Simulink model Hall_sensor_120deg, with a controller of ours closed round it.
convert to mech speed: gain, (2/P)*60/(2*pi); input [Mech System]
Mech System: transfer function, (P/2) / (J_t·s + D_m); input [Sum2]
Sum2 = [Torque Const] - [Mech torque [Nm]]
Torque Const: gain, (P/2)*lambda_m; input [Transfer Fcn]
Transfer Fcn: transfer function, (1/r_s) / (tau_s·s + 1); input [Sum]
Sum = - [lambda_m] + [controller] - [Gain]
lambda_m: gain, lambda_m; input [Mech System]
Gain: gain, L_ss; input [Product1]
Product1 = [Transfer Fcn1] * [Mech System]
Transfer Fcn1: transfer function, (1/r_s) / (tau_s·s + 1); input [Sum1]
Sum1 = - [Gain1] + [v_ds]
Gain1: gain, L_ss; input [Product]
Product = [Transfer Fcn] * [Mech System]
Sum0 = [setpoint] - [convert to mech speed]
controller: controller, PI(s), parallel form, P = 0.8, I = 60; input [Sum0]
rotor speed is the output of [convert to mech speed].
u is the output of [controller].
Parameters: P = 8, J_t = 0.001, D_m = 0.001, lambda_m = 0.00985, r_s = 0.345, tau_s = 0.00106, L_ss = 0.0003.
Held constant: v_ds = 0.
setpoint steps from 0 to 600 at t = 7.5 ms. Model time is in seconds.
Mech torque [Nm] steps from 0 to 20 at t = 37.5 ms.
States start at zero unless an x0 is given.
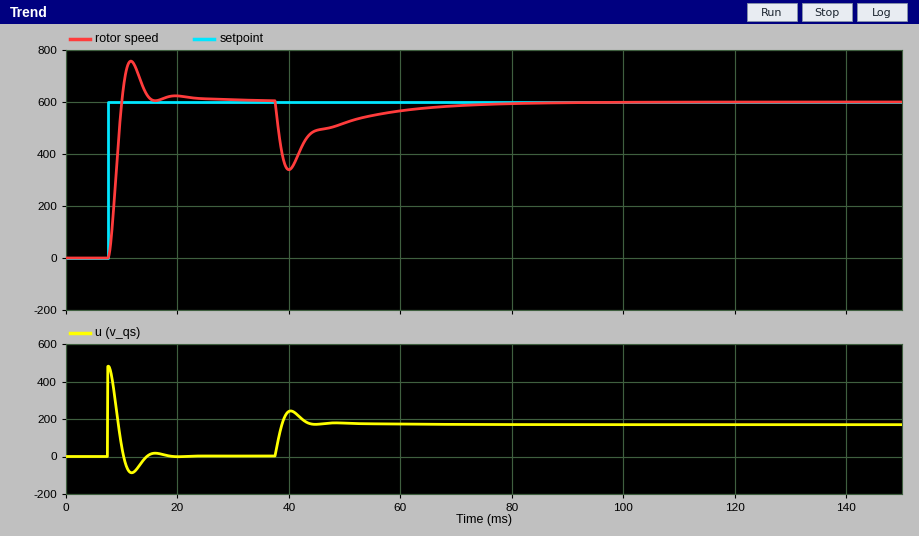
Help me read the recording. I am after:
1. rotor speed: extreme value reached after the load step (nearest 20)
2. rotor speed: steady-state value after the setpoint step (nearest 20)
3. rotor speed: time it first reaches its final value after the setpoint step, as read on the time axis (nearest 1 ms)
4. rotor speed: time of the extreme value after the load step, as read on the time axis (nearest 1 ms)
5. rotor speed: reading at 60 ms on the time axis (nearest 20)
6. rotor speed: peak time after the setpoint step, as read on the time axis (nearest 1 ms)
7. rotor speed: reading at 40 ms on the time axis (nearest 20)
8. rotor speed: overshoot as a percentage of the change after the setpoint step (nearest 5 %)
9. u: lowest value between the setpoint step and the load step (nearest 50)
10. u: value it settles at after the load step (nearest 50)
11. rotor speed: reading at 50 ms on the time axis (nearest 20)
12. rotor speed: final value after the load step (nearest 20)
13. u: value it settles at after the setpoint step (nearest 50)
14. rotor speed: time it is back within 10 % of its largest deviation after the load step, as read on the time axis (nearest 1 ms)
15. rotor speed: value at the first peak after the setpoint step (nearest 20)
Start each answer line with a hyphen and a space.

- 340
- 600
- 10 ms
- 40 ms
- 560
- 12 ms
- 340
- 25 %
- -100
- 150
- 520
- 600
- 0
- 63 ms
- 760
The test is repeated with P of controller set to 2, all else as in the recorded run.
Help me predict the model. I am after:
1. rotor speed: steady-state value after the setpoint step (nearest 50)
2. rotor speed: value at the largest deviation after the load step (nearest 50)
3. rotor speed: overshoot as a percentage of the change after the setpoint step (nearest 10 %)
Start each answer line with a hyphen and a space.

- 600
- 450
- 40 %
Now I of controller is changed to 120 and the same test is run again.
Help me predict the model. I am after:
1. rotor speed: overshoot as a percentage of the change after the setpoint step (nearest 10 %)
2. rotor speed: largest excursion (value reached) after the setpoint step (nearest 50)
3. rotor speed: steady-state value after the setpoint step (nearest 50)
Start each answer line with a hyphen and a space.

- 40 %
- 800
- 600
